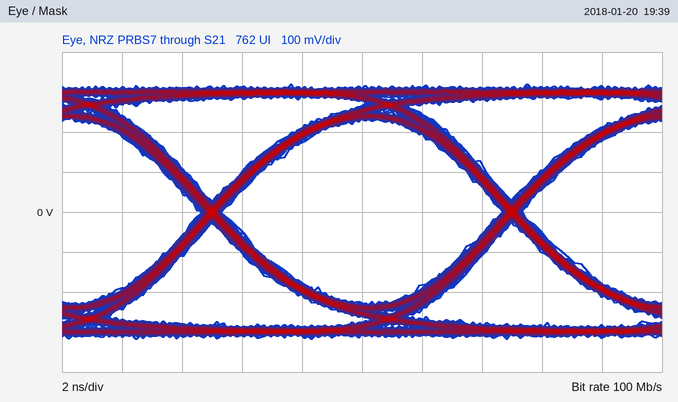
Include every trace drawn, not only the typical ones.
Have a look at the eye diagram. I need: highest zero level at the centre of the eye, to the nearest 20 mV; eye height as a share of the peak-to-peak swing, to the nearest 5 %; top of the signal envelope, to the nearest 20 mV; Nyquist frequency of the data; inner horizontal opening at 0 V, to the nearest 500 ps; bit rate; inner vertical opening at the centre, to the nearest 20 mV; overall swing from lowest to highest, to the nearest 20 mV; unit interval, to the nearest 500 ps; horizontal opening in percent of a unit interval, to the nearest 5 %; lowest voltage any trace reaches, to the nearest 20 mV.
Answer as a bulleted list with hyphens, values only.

- -220 mV
- 70 %
- 320 mV
- 50 MHz
- 9.5 ns
- 100 Mb/s
- 460 mV
- 640 mV
- 10.0 ns
- 95 %
- -320 mV
